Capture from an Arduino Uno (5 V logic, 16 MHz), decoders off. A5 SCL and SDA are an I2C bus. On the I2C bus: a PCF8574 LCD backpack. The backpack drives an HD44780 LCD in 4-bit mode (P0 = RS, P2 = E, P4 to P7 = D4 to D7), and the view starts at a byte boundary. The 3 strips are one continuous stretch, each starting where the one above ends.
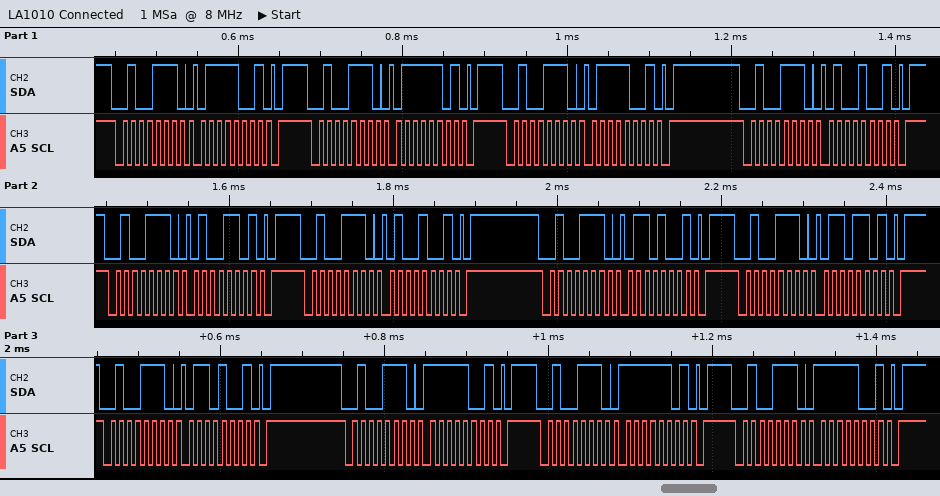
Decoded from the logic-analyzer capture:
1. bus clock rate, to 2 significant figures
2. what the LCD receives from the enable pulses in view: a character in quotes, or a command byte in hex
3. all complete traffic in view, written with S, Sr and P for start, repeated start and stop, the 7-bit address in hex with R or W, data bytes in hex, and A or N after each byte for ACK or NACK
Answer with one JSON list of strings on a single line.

["100 kHz", "'t' 'o'", "S 27W A 79 A P S 27W A 7D A P S 27W A 79 A P S 27W A 49 A P S 27W A 4D A P S 27W A 49 A P S 27W A 69 A P S 27W A 6D A P S 27W A 69 A P S 27W A F9 A P S 27W A FD A P S 27W A F9 A P"]
